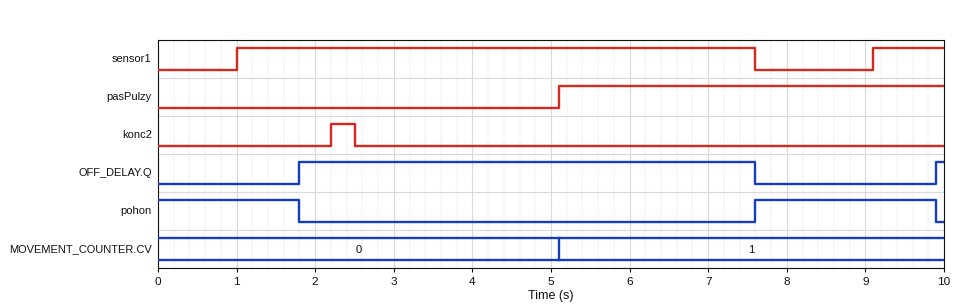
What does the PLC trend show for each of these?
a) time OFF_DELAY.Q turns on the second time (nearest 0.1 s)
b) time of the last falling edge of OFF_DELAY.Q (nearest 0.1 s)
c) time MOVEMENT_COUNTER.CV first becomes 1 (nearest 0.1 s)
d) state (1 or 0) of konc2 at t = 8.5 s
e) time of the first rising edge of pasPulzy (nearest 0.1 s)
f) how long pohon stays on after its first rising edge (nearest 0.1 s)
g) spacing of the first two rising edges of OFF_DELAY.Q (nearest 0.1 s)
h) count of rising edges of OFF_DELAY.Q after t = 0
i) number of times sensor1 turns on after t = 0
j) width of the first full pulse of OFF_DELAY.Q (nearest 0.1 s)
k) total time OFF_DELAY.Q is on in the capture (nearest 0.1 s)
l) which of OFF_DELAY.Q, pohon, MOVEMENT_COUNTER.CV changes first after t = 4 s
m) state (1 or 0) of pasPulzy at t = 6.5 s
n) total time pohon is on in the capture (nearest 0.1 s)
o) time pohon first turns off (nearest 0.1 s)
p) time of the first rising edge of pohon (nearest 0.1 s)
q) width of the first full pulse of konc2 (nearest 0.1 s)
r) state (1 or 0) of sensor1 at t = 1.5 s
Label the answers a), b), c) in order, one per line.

a) 9.9 s
b) 7.6 s
c) 5.1 s
d) 0
e) 5.1 s
f) 2.3 s
g) 8.1 s
h) 2
i) 2
j) 5.8 s
k) 5.9 s
l) MOVEMENT_COUNTER.CV
m) 1
n) 4.1 s
o) 1.8 s
p) 7.6 s
q) 0.3 s
r) 1
